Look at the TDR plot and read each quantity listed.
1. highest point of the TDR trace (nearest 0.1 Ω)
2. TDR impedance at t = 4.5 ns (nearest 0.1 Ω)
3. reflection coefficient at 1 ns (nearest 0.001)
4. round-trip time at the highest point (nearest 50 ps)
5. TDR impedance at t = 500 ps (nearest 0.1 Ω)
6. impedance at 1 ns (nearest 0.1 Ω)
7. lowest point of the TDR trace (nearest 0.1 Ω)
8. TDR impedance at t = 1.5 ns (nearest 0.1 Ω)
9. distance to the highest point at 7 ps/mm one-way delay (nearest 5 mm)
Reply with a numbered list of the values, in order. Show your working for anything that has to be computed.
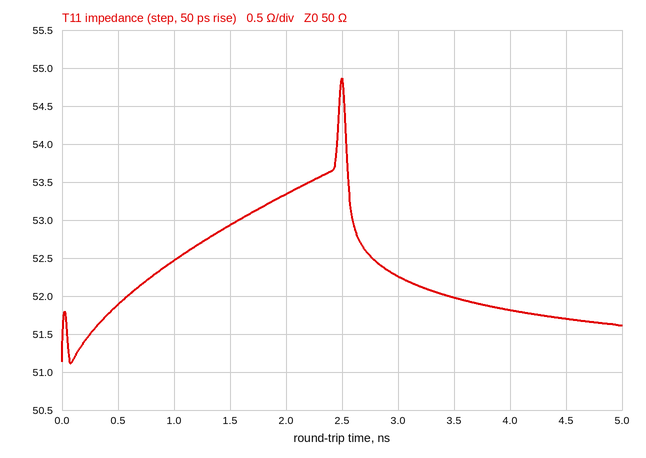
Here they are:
1. 54.9 Ω
2. 51.7 Ω
3. (52.5 − 50)/(52.5 + 50) ≈ +0.024
4. 2.50 ns
5. 51.9 Ω
6. 52.5 Ω
7. 51.1 Ω
8. 52.9 Ω
9. 2.50 ns / 2 / 7 ps/mm ≈ 179 mm, so 180 mm to the nearest 5 mm
